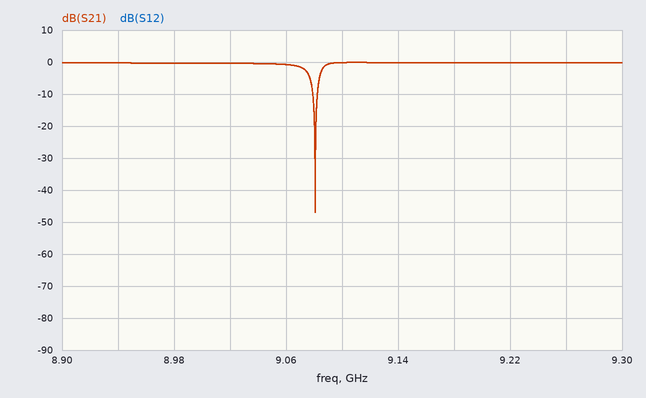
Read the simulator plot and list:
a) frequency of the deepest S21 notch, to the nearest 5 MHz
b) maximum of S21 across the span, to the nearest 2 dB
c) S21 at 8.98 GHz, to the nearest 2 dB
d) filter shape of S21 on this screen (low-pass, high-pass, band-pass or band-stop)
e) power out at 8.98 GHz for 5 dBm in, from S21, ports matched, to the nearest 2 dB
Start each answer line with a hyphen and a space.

- 9.080 GHz
- 0 dB
- 0 dB
- band-stop
- 4 dBm
